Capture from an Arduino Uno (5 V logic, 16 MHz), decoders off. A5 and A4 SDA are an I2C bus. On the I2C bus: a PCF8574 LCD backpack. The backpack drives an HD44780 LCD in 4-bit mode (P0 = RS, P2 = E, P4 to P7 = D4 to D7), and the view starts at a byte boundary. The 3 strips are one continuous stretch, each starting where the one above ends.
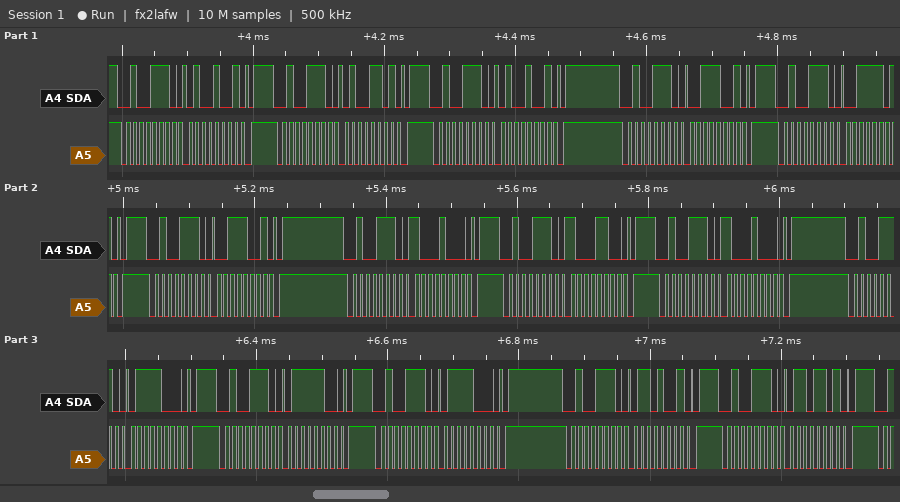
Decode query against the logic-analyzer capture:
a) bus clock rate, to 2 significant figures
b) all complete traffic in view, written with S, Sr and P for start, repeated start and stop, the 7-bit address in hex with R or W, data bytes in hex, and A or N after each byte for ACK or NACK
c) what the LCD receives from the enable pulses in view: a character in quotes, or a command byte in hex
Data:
100 kHz
S 27W A 49 A P S 27W A 4D A P S 27W A 49 A P S 27W A 39 A P S 27W A 3D A P S 27W A 39 A P S 27W A 88 A P S 27W A 8C A P S 27W A 88 A P S 27W A 78 A P S 27W A 7C A P S 27W A 78 A P S 27W A 69 A P S 27W A 6D A P
'C' 0x87
